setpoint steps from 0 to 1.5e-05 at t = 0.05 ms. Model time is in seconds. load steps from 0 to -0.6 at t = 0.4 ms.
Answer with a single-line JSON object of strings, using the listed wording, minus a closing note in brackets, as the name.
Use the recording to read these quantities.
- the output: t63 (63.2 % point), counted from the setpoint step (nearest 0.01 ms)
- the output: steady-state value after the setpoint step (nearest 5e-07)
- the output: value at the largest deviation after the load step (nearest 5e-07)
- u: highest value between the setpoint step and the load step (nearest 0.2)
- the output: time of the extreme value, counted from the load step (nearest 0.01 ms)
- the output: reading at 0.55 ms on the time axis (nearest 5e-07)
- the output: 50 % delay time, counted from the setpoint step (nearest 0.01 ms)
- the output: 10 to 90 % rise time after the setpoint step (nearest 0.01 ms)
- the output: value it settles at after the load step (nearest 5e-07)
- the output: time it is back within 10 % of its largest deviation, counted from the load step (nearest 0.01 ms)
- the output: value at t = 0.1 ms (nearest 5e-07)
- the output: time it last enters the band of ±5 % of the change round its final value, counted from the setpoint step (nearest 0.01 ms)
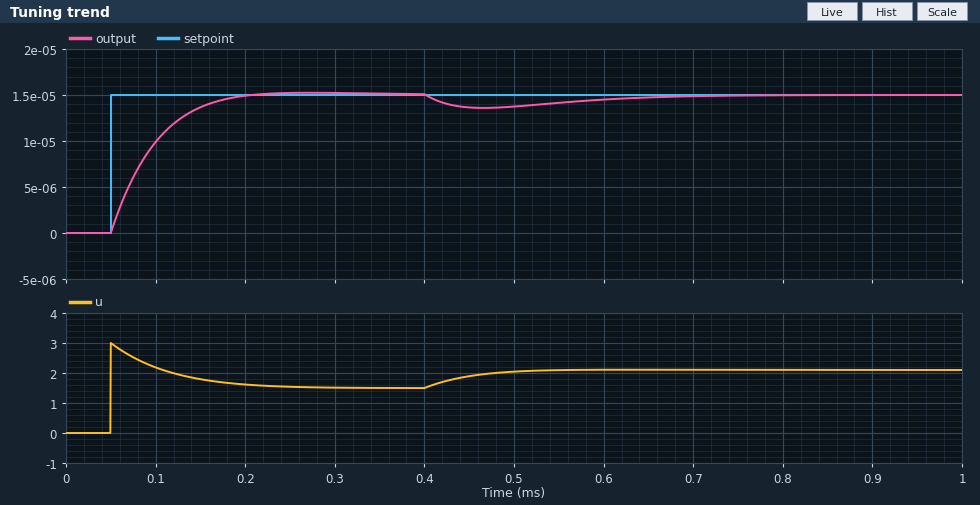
{"the output: t63 (63.2 % point), counted from the setpoint step": "0.05 ms", "the output: steady-state value after the setpoint step": "0.0000150", "the output: value at the largest deviation after the load step": "0.0000135", "u: highest value between the setpoint step and the load step": "3.0", "the output: time of the extreme value, counted from the load step": "0.07 ms", "the output: reading at 0.55 ms on the time axis": "0.0000140", "the output: 50 % delay time, counted from the setpoint step": "0.03 ms", "the output: 10 to 90 % rise time after the setpoint step": "0.09 ms", "the output: value it settles at after the load step": "0.0000150", "the output: time it is back within 10 % of its largest deviation, counted from the load step": "0.29 ms", "the output: value at t = 0.1 ms": "0.0000100", "the output: time it last enters the band of ±5 % of the change round its final value, counted from the setpoint step": "0.12 ms"}
